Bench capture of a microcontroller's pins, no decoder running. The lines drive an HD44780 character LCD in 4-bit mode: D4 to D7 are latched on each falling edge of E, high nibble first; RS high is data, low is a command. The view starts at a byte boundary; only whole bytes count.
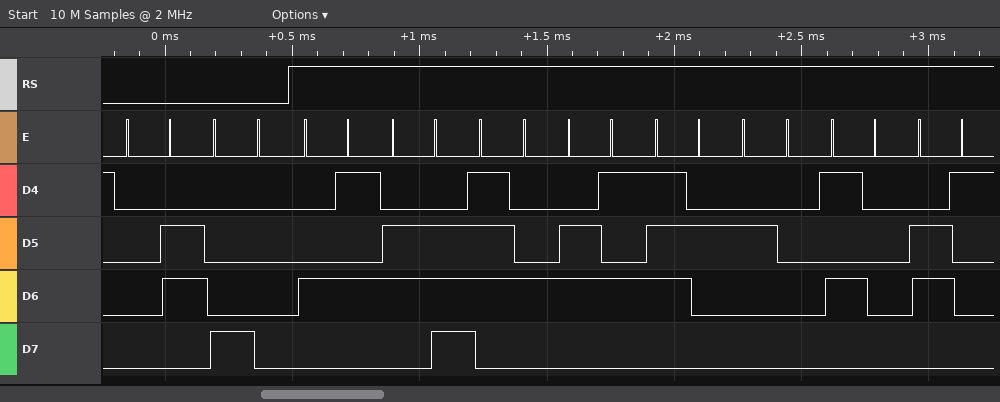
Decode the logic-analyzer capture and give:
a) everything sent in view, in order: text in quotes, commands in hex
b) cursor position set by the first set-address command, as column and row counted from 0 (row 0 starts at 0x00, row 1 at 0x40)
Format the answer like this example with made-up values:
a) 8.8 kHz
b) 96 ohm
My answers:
a) 0x06 0x80 "Enter Pa"
b) column 0, row 0
